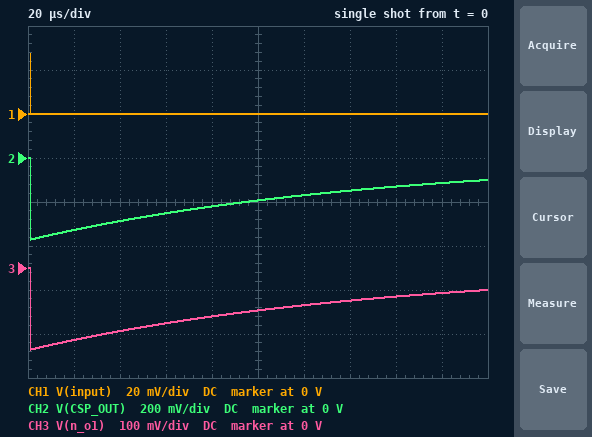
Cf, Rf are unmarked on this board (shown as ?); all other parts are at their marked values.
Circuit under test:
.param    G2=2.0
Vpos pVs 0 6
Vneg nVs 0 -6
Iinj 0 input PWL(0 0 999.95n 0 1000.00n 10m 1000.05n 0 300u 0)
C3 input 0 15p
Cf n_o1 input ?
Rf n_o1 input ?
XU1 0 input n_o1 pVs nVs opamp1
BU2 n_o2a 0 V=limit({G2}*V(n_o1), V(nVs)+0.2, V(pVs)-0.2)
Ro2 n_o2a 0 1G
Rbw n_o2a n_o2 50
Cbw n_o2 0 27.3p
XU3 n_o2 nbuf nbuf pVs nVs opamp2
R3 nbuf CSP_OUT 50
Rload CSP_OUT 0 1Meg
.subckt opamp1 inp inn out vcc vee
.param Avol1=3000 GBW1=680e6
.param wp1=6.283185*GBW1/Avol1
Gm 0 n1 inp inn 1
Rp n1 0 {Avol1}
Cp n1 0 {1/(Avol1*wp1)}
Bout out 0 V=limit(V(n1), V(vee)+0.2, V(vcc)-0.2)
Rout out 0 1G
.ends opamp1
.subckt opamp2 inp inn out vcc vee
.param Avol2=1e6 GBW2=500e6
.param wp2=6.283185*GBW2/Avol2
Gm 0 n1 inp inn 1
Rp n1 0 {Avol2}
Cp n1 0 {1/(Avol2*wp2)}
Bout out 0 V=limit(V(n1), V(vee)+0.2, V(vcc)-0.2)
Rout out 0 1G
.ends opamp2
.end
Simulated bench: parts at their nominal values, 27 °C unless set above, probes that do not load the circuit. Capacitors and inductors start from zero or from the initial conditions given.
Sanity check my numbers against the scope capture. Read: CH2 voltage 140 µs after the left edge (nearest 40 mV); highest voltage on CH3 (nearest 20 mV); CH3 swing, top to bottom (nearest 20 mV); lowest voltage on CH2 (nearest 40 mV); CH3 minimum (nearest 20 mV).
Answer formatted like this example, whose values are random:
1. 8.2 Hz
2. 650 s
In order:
1. -160 mV
2. 0 V
3. 180 mV
4. -360 mV
5. -180 mV
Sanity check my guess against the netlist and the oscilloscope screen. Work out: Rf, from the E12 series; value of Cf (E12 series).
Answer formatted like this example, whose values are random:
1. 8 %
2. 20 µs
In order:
1. 56 MΩ
2. 2.7 pF
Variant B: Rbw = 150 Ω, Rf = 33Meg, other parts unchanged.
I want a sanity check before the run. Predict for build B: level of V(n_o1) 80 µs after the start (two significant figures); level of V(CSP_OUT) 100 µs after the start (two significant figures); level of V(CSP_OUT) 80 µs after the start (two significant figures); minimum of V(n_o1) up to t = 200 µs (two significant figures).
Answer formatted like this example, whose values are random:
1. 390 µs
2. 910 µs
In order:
1. -77 mV
2. -120 mV
3. -150 mV
4. -190 mV
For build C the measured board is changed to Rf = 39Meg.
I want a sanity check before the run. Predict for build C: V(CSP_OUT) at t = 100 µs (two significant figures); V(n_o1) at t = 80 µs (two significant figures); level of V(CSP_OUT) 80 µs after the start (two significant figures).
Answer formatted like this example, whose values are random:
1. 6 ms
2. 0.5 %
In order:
1. -150 mV
2. -88 mV
3. -180 mV
